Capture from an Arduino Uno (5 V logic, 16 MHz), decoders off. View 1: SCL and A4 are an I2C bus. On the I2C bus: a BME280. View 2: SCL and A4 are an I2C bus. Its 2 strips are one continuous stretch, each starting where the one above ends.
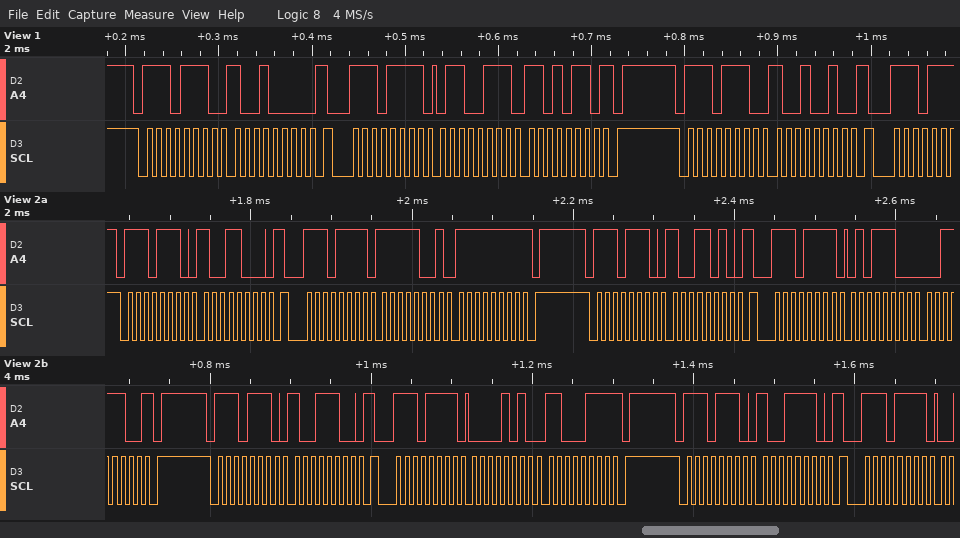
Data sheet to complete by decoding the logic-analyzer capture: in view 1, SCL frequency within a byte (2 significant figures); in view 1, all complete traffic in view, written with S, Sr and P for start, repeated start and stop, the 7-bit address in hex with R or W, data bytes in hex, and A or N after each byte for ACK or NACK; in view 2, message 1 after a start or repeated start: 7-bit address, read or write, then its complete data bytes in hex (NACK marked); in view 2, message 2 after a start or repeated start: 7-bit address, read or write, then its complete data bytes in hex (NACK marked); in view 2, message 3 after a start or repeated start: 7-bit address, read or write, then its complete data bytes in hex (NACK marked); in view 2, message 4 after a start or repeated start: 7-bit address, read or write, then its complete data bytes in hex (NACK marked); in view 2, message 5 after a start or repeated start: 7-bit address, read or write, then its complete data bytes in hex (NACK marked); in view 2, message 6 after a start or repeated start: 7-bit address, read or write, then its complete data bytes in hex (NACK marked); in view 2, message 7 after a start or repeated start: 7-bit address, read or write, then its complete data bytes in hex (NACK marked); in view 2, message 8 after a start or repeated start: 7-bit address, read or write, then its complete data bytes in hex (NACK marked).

100 kHz
S 77W A 90 A Sr 77R A 67 A D6 N P S 77W A 92 A
0x77 write: 98
0x77 read: F9 FF NACK
0x77 write: 9A
0x77 read: 5C 3C NACK
0x77 write: 9C
0x77 read: 0A C7 NACK
0x77 write: 9E
0x77 read
